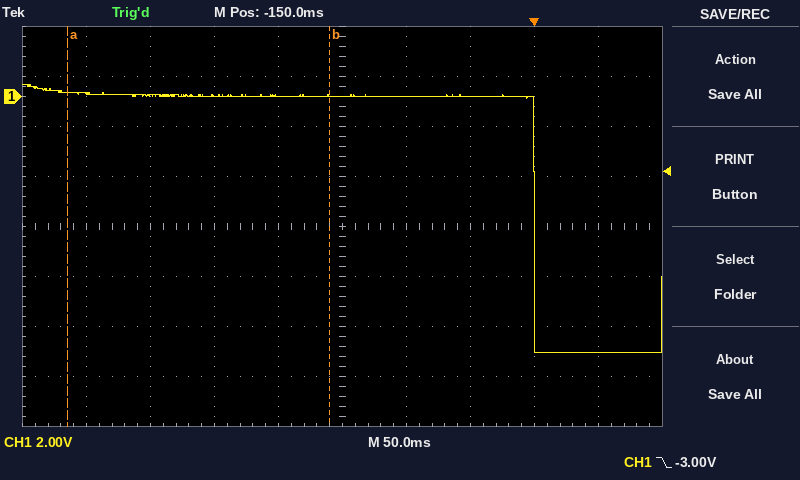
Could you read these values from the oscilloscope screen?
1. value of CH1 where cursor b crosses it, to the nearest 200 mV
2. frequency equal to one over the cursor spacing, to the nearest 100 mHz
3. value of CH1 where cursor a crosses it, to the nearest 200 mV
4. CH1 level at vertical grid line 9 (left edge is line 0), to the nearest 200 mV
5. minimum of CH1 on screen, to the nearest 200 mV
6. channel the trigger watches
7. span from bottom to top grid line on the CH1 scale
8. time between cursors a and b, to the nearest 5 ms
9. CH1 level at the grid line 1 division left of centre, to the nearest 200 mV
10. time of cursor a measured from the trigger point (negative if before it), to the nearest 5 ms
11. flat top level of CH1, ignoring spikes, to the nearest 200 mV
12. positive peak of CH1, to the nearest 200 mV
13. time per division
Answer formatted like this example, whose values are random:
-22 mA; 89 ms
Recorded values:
0.0 V; 4.9 Hz; 200 mV; -10.2 V; -10.2 V; CH1; 16 V; 205 ms; 0.0 V; -365 ms; 0.0 V; 400 mV; 50 ms
